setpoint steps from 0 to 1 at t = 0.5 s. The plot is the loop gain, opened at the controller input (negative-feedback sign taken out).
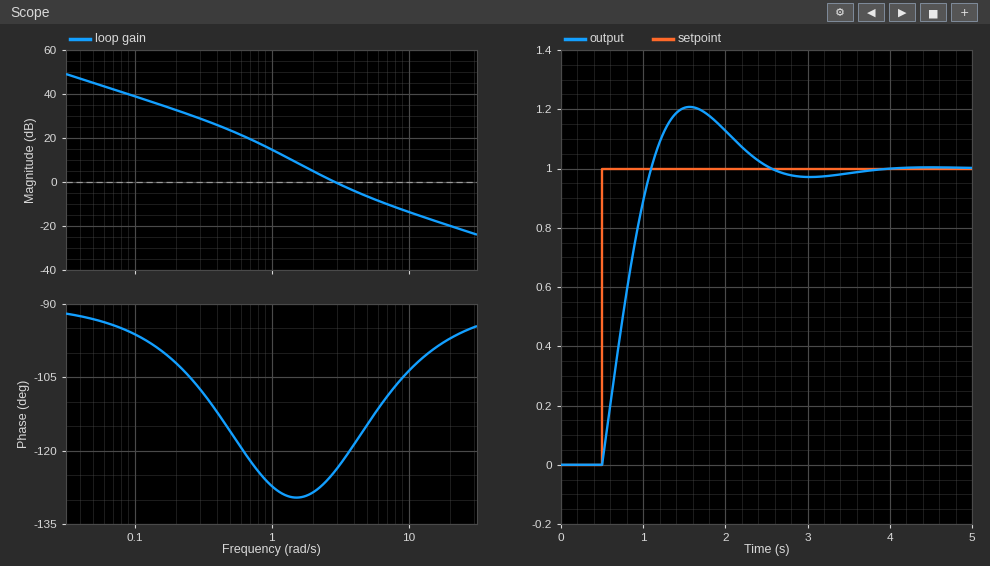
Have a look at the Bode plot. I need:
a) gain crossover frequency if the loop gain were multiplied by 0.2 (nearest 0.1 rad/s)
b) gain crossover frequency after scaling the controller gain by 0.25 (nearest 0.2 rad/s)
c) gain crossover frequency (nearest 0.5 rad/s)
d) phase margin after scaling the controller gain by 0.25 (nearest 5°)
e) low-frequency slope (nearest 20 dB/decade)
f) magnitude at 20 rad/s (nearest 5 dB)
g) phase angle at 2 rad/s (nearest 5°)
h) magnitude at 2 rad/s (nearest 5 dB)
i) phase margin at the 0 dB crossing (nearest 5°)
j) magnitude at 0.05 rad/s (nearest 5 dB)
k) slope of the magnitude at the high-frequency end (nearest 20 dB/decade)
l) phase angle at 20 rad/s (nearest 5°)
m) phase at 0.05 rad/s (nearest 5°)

1.1 rad/s
1.2 rad/s
3.0 rad/s
50°
-20 dB/decade
-20 dB
-130°
5 dB
55°
45 dB
-20 dB/decade
-95°
-95°
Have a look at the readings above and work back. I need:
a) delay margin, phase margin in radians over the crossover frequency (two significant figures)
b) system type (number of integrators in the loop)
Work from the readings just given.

0.32 s
1
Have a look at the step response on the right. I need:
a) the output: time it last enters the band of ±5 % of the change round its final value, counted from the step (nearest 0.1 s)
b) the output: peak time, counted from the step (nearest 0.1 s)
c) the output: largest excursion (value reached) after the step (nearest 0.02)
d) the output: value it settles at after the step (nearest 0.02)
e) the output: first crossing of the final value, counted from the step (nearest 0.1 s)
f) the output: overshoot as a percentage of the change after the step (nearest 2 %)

1.8 s
1.1 s
1.20
1.00
0.6 s
20 %
